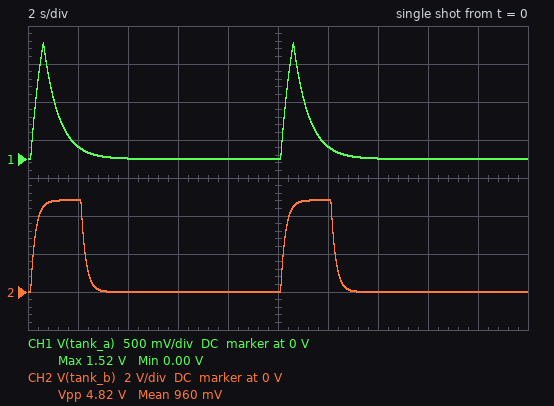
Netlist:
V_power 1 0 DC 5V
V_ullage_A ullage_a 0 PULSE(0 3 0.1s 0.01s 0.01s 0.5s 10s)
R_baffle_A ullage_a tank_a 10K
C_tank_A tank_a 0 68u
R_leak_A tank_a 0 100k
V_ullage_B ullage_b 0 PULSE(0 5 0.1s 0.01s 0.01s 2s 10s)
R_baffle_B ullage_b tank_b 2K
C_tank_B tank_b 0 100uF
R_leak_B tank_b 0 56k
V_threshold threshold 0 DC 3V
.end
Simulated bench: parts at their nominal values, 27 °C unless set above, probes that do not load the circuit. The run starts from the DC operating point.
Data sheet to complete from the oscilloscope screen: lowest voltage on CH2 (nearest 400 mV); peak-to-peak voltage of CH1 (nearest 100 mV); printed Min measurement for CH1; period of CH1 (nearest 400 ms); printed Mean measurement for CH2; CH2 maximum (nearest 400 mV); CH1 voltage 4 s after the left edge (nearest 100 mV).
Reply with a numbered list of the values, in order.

1. 0 V
2. 1.5 V
3. 0.00 V
4. 10.0 s
5. 960 mV
6. 4.8 V
7. 0 V
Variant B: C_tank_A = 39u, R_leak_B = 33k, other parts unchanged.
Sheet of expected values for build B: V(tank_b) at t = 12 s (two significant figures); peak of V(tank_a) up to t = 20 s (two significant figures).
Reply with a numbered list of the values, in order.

1. 4.7 V
2. 2.1 V
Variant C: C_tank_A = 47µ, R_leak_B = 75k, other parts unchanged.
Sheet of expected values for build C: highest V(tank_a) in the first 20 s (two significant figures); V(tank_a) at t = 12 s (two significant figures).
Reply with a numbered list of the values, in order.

1. 1.9 V
2. 74 mV
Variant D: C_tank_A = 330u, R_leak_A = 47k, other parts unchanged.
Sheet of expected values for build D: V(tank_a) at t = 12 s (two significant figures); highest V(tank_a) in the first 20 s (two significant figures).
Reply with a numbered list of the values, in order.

1. 260 mV
2. 430 mV
